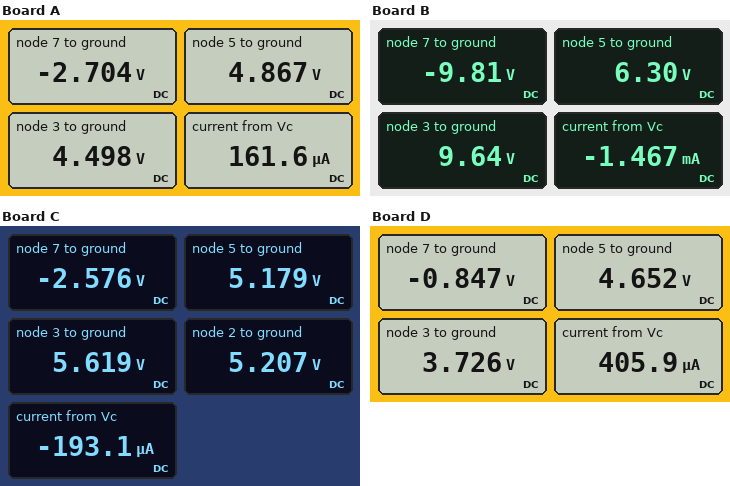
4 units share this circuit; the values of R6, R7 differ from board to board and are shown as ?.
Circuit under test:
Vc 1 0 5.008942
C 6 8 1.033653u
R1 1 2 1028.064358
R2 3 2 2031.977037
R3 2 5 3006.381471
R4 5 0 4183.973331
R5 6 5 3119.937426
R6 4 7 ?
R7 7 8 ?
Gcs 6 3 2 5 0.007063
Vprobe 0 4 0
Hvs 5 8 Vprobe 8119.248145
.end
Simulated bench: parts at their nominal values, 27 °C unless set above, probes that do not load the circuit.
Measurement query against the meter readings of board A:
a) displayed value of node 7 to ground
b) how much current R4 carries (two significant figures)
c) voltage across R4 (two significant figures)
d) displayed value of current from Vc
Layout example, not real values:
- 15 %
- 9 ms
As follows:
- -2.704 V
- 1.2 mA
- 4.9 V
- 161.6 µA
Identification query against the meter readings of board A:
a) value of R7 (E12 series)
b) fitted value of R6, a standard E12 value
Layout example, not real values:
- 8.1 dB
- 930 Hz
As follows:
- 560 Ω
- 2.7 kΩ
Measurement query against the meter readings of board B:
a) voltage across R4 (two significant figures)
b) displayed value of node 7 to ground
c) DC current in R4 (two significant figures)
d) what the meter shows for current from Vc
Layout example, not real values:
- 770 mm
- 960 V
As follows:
- 6.3 V
- -9.81 V
- 1.5 mA
- -1.467 mA
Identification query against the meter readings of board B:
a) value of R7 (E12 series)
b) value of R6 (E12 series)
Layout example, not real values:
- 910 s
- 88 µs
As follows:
- 2.7 kΩ
- 3.3 kΩ
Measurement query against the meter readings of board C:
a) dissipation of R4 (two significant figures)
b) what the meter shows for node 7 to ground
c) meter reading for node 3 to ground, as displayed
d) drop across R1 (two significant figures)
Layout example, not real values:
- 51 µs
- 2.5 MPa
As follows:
- 6.4 mW
- -2.576 V
- 5.619 V
- 200 mV
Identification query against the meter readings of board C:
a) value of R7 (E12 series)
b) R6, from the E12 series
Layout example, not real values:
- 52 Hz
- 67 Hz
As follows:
- 2.7 kΩ
- 1.8 kΩ
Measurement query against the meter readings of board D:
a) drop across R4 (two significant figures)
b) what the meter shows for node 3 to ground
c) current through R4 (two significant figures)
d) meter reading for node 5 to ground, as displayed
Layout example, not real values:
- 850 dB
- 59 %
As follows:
- 4.7 V
- 3.726 V
- 1.1 mA
- 4.652 V
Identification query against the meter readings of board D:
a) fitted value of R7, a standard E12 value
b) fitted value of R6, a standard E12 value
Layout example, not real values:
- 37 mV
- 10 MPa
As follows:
- 330 Ω
- 1.2 kΩ
